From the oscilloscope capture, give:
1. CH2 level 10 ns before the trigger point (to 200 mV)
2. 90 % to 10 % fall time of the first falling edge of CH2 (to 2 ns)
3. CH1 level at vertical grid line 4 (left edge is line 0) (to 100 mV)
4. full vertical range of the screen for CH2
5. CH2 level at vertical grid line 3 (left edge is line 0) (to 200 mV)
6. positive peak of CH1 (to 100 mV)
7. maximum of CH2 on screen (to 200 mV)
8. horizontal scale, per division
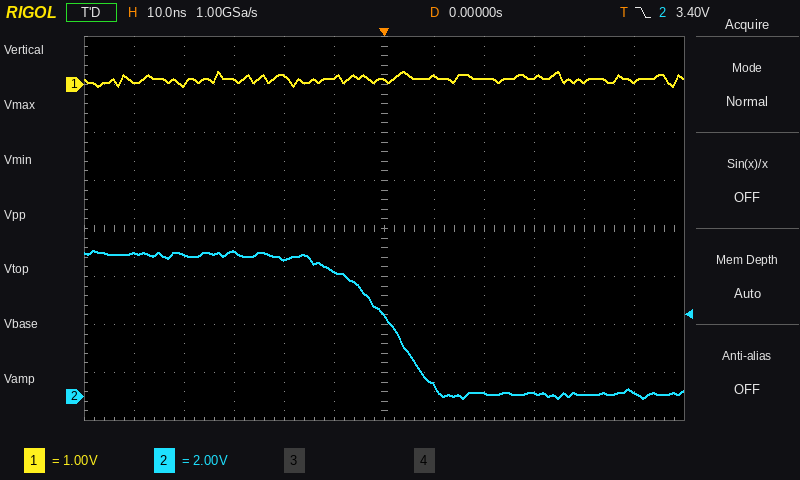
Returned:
5.2 V
20 ns
200 mV
16 V
6.0 V
300 mV
6.0 V
10 ns
